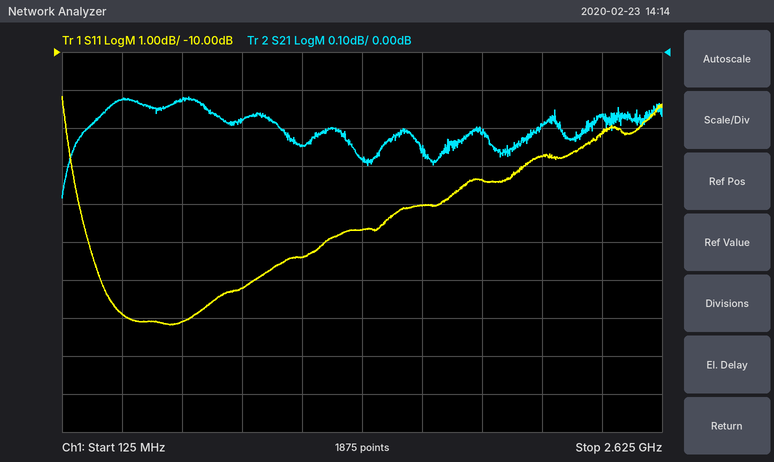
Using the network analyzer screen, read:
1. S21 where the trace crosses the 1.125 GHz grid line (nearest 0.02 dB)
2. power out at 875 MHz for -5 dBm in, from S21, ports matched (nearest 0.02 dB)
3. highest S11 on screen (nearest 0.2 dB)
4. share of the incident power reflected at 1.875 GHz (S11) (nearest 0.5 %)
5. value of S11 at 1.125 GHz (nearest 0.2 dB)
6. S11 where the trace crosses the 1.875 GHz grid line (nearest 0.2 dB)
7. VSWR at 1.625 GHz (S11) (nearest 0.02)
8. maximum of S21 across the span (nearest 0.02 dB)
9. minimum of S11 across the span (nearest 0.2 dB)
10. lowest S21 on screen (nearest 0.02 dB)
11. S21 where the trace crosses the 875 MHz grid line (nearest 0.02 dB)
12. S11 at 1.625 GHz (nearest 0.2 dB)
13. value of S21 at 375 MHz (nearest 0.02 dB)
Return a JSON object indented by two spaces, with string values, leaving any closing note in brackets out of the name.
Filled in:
{
  "S21 where the trace crosses the 1.125 GHz grid line": "-0.24 dB",
  "power out at 875 MHz for -5 dBm in, from S21, ports matched": "-5.18 dBm",
  "highest S11 on screen": "-11.2 dB",
  "share of the incident power reflected at 1.875 GHz (S11)": "4.5 %",
  "value of S11 at 1.125 GHz": "-15.4 dB",
  "S11 where the trace crosses the 1.875 GHz grid line": "-13.4 dB",
  "VSWR at 1.625 GHz (S11)": "1.50",
  "maximum of S21 across the span": "-0.12 dB",
  "minimum of S11 across the span": "-17.2 dB",
  "lowest S21 on screen": "-0.38 dB",
  "S21 where the trace crosses the 875 MHz grid line": "-0.18 dB",
  "S11 at 1.625 GHz": "-14.0 dB",
  "value of S21 at 375 MHz": "-0.12 dB"
}
